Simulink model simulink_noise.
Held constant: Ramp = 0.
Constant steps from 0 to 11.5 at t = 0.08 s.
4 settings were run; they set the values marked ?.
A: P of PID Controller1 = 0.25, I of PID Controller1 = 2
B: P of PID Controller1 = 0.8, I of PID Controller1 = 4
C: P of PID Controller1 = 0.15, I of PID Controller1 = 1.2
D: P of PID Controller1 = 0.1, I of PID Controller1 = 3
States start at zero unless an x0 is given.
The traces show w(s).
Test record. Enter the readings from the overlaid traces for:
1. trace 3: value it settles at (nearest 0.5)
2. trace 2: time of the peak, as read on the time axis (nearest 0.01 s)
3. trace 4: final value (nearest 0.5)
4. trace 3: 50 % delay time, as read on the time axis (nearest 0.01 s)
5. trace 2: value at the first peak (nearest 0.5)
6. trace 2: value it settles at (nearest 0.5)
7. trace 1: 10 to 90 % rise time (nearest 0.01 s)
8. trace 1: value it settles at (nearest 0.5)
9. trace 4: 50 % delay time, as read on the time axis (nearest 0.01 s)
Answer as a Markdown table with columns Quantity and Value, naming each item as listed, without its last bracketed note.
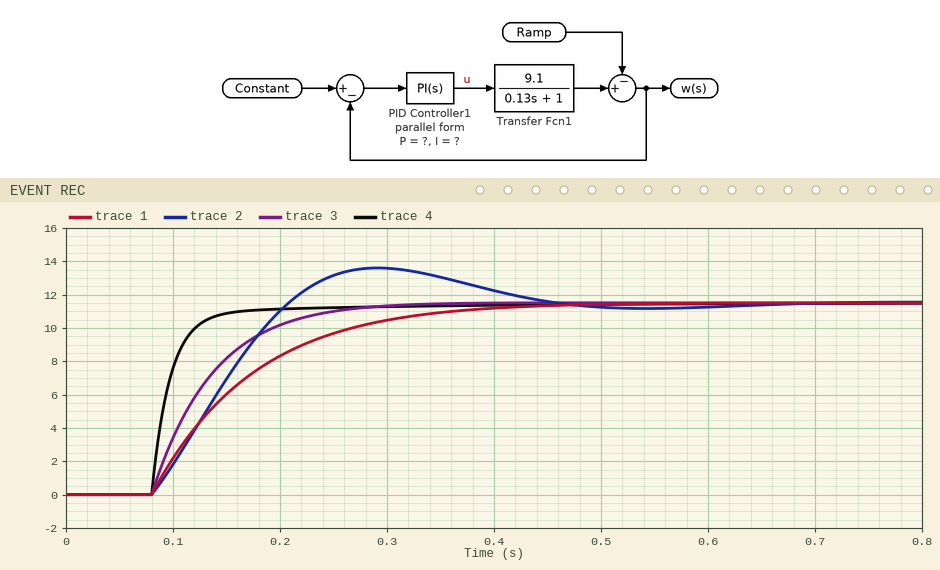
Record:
| Quantity | Value |
|---|---|
| trace 3: value it settles at | 11.5 |
| trace 2: time of the peak, as read on the time axis | 0.29 s |
| trace 4: final value | 11.5 |
| trace 3: 50 % delay time, as read on the time axis | 0.12 s |
| trace 2: value at the first peak | 13.5 |
| trace 2: value it settles at | 11.5 |
| trace 1: 10 to 90 % rise time | 0.20 s |
| trace 1: value it settles at | 11.5 |
| trace 4: 50 % delay time, as read on the time axis | 0.09 s |
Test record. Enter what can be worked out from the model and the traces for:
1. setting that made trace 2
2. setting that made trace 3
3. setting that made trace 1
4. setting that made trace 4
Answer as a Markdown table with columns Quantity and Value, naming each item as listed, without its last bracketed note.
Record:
| Quantity | Value |
|---|---|
| setting that made trace 2 | D |
| setting that made trace 3 | A |
| setting that made trace 1 | C |
| setting that made trace 4 | B |
